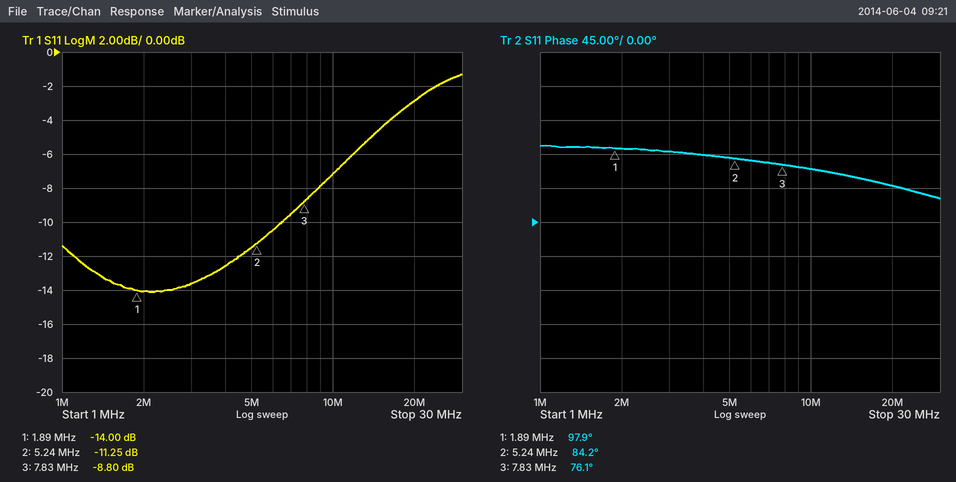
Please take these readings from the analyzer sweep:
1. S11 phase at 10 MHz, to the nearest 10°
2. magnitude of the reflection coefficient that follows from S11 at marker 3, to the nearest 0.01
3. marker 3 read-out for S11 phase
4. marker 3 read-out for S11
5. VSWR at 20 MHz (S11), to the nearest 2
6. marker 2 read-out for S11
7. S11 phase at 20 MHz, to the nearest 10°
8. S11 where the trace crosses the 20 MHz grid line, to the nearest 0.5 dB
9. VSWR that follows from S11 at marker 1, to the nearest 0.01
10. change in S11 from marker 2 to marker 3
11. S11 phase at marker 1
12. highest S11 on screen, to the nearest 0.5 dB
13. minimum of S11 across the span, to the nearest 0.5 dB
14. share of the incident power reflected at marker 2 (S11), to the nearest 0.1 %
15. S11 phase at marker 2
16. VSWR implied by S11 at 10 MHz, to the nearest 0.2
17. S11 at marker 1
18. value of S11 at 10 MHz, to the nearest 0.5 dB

70°
0.36
76.1°
-8.80 dB
6
-11.25 dB
50°
-3.0 dB
1.50
2.45 dB
97.9°
-1.5 dB
-14.0 dB
7.5 %
84.2°
2.6
-14.00 dB
-7.0 dB
